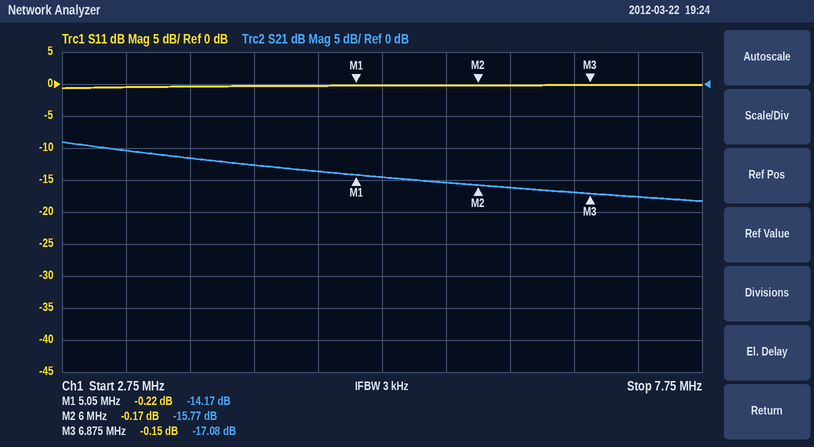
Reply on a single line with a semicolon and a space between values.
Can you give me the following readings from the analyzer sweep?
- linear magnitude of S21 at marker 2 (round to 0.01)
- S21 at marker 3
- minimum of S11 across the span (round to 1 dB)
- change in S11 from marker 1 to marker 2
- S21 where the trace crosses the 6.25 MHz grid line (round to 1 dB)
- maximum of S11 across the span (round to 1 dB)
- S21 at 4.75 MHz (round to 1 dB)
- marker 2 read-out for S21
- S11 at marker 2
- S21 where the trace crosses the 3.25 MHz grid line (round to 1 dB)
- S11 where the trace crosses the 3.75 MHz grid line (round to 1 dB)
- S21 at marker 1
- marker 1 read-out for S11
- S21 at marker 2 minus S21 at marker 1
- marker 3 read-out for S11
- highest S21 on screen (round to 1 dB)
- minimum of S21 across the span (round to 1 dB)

0.16; -17.08 dB; -1 dB; 0.05 dB; -16 dB; 0 dB; -14 dB; -15.77 dB; -0.17 dB; -10 dB; 0 dB; -14.17 dB; -0.22 dB; -1.60 dB; -0.15 dB; -9 dB; -18 dB
